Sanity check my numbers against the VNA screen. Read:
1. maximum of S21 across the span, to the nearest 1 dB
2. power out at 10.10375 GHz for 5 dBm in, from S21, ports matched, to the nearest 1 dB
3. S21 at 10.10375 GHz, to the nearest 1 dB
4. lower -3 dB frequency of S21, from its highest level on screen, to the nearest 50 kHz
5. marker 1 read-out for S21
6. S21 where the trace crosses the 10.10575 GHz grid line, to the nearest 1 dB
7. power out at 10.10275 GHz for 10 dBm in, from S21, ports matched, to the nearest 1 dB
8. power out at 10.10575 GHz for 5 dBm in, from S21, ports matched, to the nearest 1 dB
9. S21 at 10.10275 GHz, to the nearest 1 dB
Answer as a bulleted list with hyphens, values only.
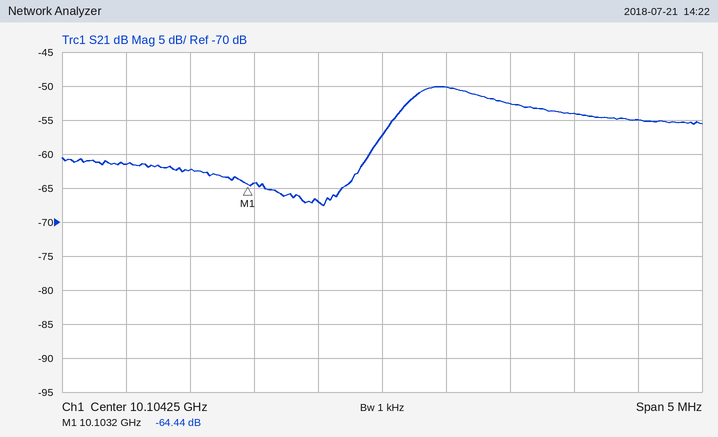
- -50 dB
- -62 dBm
- -67 dB
- 10.10440 GHz
- -64.44 dB
- -54 dB
- -52 dBm
- -49 dBm
- -62 dB
